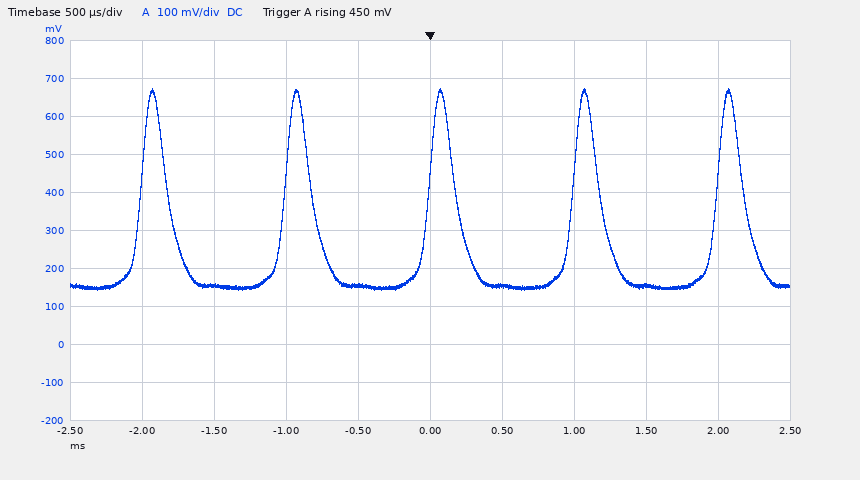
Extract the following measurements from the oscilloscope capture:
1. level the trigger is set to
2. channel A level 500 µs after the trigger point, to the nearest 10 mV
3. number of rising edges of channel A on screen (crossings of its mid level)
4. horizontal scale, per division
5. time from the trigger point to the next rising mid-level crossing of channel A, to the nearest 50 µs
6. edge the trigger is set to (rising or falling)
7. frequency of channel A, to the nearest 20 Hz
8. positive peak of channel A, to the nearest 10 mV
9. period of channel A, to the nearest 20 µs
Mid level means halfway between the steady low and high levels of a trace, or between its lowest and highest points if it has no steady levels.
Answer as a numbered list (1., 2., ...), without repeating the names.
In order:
1. 450 mV
2. 160 mV
3. 5
4. 500 µs
5. 1.00 ms
6. rising
7. 1.00 kHz
8. 670 mV
9. 1.00 ms
